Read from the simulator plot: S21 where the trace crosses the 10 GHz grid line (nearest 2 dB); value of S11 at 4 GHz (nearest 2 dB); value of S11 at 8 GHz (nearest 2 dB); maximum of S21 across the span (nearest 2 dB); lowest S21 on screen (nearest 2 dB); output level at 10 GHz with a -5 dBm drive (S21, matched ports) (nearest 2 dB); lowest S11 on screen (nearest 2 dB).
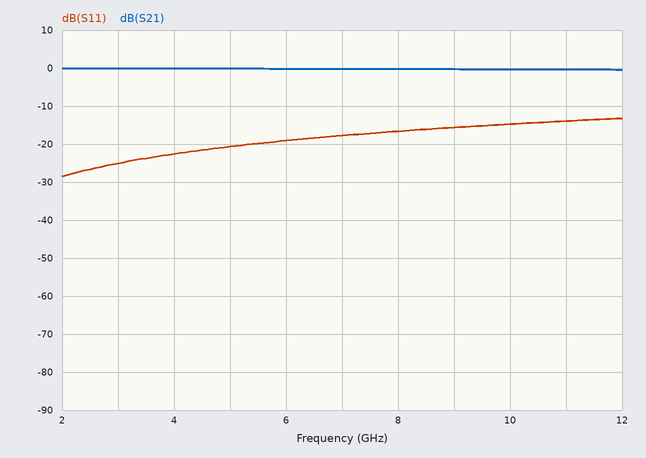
0 dB
-22 dB
-16 dB
0 dB
0 dB
-6 dBm
-28 dB
